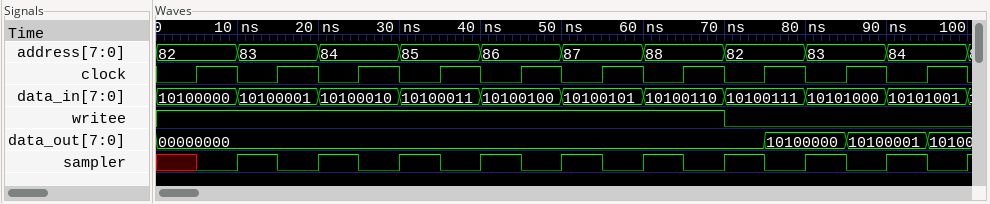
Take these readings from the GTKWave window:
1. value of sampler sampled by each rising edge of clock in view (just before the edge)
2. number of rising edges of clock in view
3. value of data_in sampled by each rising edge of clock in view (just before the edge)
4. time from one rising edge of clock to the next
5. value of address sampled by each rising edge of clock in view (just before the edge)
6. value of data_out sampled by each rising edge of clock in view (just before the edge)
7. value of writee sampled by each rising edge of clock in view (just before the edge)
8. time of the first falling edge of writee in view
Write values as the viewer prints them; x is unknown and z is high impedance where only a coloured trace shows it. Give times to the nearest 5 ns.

x 1 1 1 1 1 1 1 1 1
10
10100000, 10100001, 10100010, 10100011, 10100100, 10100101, 10100110, 10100111, 10101000, 10101001
10 ns
82, 83, 84, 85, 86, 87, 88, 82, 83, 84
00000000, 00000000, 00000000, 00000000, 00000000, 00000000, 00000000, 00000000, 10100000, 10100001
1 1 1 1 1 1 1 0 0 0
70 ns
